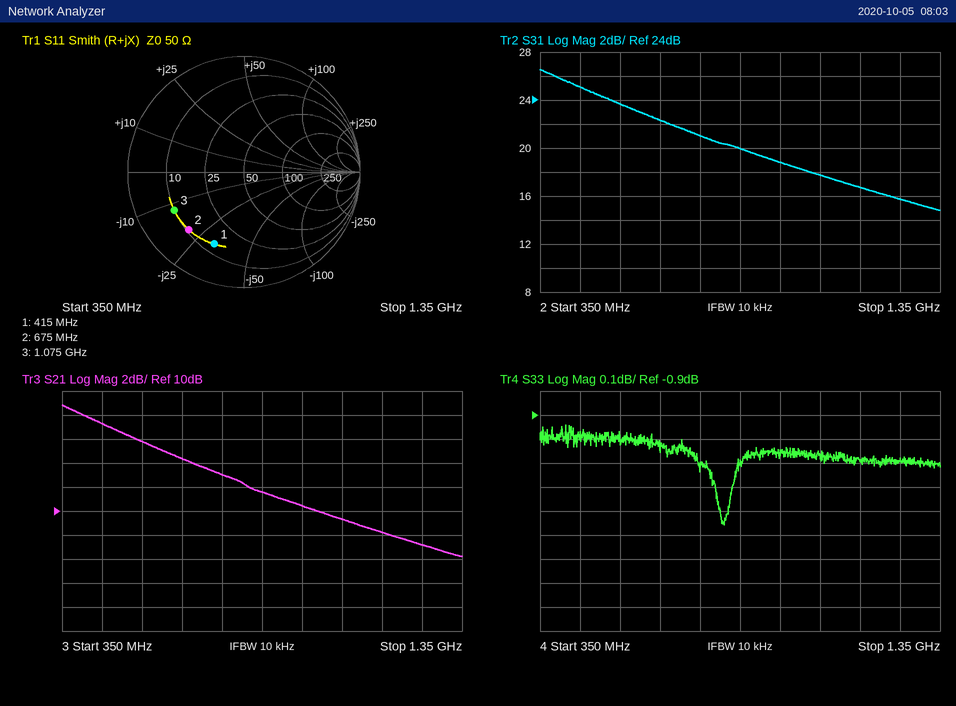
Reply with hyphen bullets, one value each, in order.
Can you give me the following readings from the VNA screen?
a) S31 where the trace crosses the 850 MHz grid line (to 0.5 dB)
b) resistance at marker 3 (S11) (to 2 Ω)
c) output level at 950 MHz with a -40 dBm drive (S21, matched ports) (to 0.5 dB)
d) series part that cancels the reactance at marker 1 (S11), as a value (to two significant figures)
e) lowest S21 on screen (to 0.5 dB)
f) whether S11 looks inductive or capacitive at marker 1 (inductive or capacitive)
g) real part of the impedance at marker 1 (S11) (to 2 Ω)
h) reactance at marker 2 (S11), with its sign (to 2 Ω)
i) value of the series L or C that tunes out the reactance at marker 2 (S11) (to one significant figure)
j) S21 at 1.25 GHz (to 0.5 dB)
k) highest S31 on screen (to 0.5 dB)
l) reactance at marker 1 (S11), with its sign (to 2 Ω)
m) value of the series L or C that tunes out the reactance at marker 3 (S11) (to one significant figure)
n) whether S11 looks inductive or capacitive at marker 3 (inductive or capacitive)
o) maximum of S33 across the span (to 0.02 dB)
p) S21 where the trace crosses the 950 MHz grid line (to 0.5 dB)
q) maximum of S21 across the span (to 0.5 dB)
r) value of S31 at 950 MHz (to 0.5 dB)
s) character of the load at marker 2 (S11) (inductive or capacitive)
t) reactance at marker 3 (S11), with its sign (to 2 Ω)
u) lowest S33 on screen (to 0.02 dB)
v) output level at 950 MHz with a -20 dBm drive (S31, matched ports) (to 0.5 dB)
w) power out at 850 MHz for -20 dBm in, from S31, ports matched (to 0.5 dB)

- 20.0 dB
- 10 Ω
- -29.5 dBm
- 12 nH
- 6.0 dB
- capacitive
- 14 Ω
- -20 Ω
- 5 nH
- 7.0 dB
- 26.5 dB
- -32 Ω
- 2 nH
- capacitive
- -0.94 dB
- 10.5 dB
- 19.0 dB
- 19.0 dB
- capacitive
- -12 Ω
- -1.36 dB
- -1.0 dBm
- 0.0 dBm
